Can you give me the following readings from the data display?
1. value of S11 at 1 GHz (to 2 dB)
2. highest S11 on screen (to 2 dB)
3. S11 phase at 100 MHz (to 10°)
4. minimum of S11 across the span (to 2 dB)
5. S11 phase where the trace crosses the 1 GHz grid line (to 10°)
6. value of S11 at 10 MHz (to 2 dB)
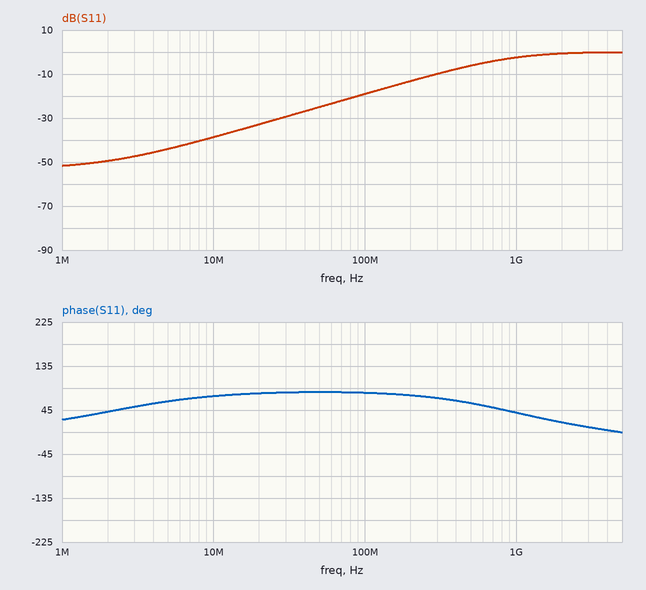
-2 dB
0 dB
80°
-52 dB
40°
-38 dB
